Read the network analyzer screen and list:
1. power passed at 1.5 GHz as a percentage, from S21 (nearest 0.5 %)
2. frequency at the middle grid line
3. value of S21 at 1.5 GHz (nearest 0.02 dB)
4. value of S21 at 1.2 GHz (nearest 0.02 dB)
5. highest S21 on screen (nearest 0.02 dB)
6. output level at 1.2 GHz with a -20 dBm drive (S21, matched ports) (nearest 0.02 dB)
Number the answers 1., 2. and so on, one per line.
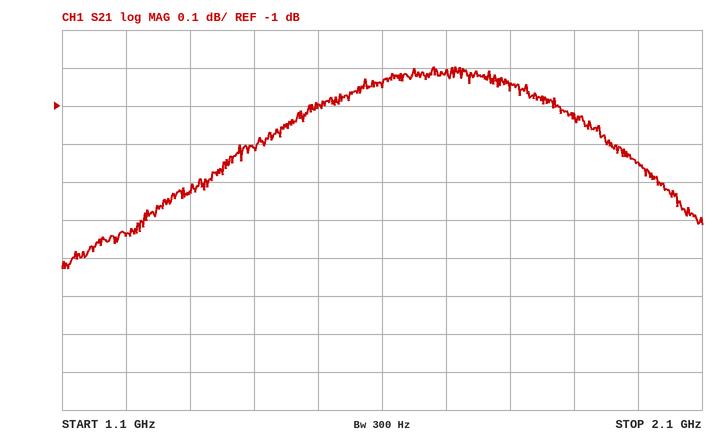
1. 79.5 %
2. 1.6 GHz
3. -1.00 dB
4. -1.34 dB
5. -0.90 dB
6. -21.34 dBm
